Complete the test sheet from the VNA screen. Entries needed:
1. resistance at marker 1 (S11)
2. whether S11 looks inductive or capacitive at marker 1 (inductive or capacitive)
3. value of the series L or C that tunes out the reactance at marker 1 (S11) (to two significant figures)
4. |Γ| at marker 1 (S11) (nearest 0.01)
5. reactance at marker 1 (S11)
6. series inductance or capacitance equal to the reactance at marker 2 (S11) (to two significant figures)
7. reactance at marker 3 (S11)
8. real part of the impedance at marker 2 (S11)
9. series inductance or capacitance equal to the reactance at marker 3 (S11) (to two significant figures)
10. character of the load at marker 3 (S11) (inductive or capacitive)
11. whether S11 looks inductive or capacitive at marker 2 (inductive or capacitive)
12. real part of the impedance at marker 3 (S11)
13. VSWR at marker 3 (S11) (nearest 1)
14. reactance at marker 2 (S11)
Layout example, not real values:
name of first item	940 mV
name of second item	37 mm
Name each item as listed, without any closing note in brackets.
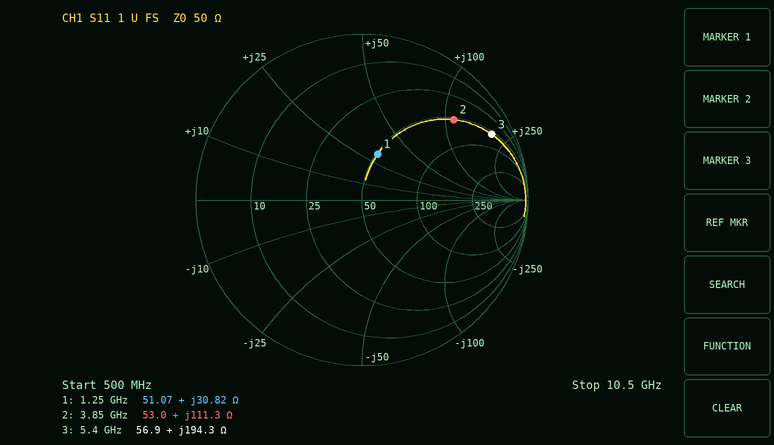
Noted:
resistance at marker 1	51.07 Ω
whether S11 looks inductive or capacitive at marker 1	inductive
value of the series L or C that tunes out the reactance at marker 1 (S11)	4.1 pF
|Γ| at marker 1 (S11)	0.29
reactance at marker 1	+30.82 Ω
series inductance or capacitance equal to the reactance at marker 2 (S11)	4.6 nH
reactance at marker 3	+194.3 Ω
real part of the impedance at marker 2	53.0 Ω
series inductance or capacitance equal to the reactance at marker 3 (S11)	5.7 nH
character of the load at marker 3 (S11)	inductive
whether S11 looks inductive or capacitive at marker 2	inductive
real part of the impedance at marker 3	56.9 Ω
VSWR at marker 3 (S11)	15
reactance at marker 2	+111.3 Ω
